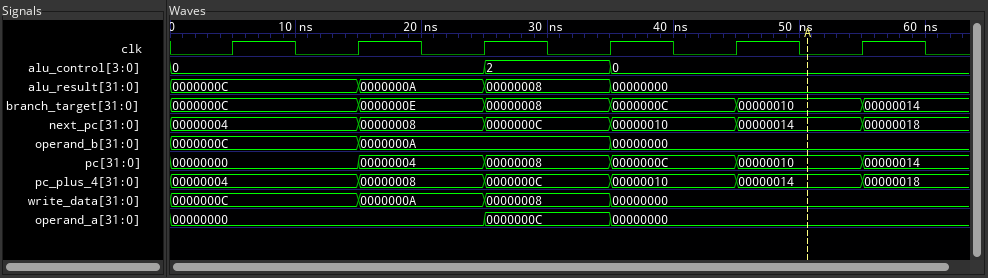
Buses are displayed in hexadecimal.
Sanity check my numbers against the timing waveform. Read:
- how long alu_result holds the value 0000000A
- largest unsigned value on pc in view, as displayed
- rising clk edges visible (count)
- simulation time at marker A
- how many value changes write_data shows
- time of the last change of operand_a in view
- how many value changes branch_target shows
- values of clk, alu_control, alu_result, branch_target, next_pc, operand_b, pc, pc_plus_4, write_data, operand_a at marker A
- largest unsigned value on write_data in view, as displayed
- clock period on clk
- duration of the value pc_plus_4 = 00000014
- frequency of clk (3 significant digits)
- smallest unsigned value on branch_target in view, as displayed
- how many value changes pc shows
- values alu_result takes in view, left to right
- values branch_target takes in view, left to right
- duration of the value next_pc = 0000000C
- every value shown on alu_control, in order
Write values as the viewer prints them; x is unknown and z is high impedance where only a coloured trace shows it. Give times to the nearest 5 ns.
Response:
10 ns
00000014
6
50 ns
3
35 ns
5
clk=0, alu_control=0, alu_result=00000000, branch_target=00000010, next_pc=00000014, operand_b=00000000, pc=00000010, pc_plus_4=00000014, write_data=00000000, operand_a=00000000
0000000C
10 ns
10 ns
100 MHz
00000008
5
0000000C, 0000000A, 00000008, 00000000
0000000C, 0000000E, 00000008, 0000000C, 00000010, 00000014
10 ns
0, 2, 0
